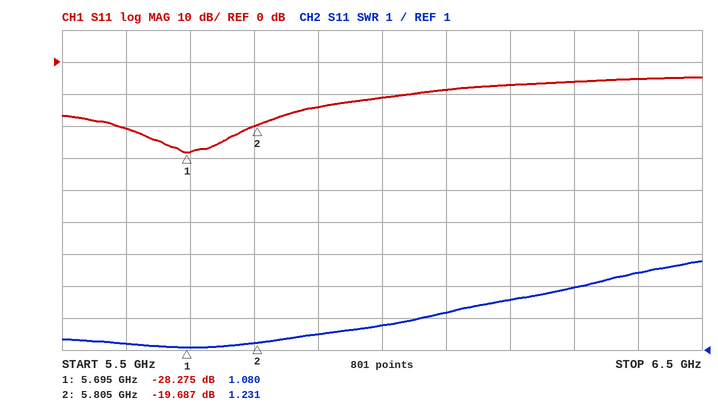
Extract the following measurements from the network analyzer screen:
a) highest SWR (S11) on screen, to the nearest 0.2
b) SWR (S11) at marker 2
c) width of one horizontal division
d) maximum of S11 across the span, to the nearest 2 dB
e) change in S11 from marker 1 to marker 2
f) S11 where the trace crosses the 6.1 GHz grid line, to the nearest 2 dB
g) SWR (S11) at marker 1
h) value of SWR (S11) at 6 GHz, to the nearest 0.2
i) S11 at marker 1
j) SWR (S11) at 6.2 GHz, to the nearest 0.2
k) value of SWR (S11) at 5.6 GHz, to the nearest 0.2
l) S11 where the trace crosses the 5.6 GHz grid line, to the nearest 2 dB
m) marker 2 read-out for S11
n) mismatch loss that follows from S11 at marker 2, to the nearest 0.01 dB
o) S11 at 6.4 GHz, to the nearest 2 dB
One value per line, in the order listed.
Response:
3.8
1.231
100 MHz
-4 dB
8.588 dB
-8 dB
1.080
1.8
-28.275 dB
2.6
1.2
-20 dB
-19.687 dB
0.05 dB
-6 dB
